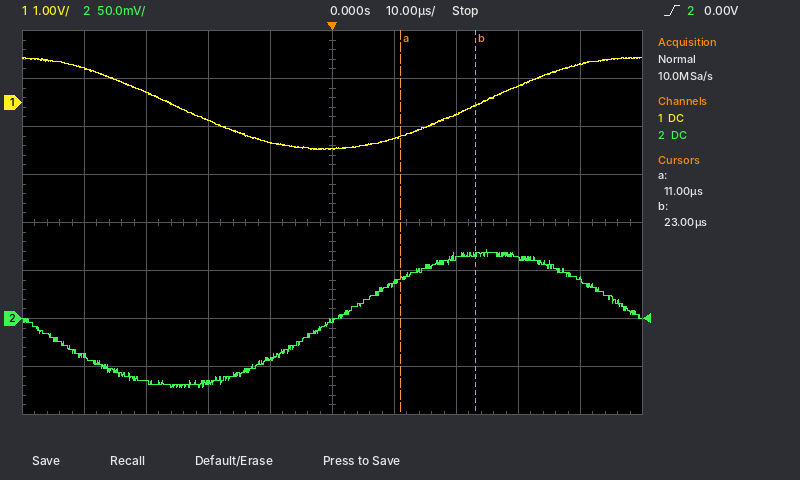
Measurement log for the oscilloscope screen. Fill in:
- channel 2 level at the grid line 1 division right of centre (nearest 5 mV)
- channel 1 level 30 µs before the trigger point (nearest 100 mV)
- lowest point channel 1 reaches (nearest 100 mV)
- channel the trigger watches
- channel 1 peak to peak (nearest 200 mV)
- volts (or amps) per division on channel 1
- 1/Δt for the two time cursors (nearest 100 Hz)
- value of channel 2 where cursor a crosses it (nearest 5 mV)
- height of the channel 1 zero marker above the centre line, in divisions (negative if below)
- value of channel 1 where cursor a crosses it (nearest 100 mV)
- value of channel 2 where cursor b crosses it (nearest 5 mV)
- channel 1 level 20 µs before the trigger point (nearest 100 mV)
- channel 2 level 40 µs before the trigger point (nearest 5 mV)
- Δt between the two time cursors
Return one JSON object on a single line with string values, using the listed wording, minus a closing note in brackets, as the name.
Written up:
{"channel 2 level at the grid line 1 division right of centre": "35 mV", "channel 1 level 30 µs before the trigger point": "200 mV", "lowest point channel 1 reaches": "-1.0 V", "channel the trigger watches": "channel 2", "channel 1 peak to peak": "2.0 V", "volts (or amps) per division on channel 1": "1 V", "1/Δt for the two time cursors": "83.3 kHz", "value of channel 2 where cursor a crosses it": "40 mV", "height of the channel 1 zero marker above the centre line, in divisions": "+2.5 div", "value of channel 1 where cursor a crosses it": "-700 mV", "value of channel 2 where cursor b crosses it": "65 mV", "channel 1 level 20 µs before the trigger point": "-400 mV", "channel 2 level 40 µs before the trigger point": "-40 mV", "Δt between the two time cursors": "12 µs"}
